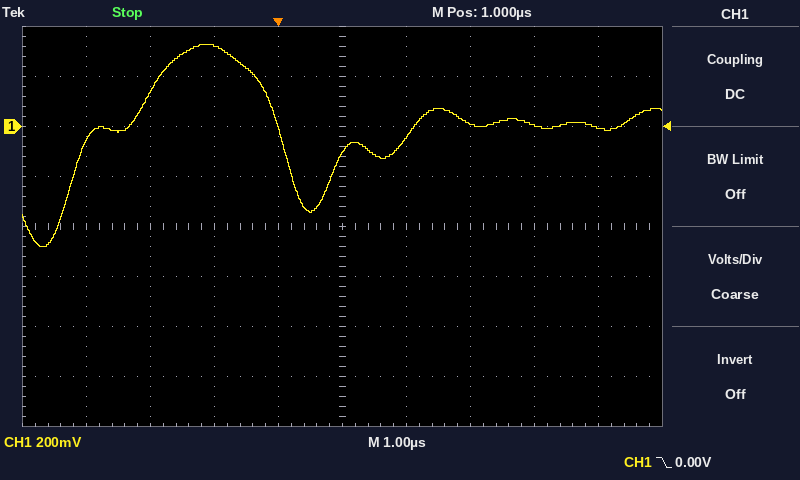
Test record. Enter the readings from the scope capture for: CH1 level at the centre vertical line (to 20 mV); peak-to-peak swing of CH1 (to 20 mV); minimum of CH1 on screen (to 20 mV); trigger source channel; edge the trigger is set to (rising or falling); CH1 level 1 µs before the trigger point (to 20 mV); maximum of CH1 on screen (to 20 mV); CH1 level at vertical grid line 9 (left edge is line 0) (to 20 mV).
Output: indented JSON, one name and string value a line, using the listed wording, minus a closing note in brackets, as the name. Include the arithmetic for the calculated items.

{
  "CH1 level at the centre vertical line": "-100 mV",
  "peak-to-peak swing of CH1": "320 mV − (-480 mV) = 800 mV",
  "minimum of CH1 on screen": "-480 mV",
  "trigger source channel": "CH1",
  "edge the trigger is set to": "falling",
  "CH1 level 1 µs before the trigger point": "320 mV",
  "maximum of CH1 on screen": "320 mV",
  "CH1 level at vertical grid line 9 (left edge is line 0)": "0 mV"
}
